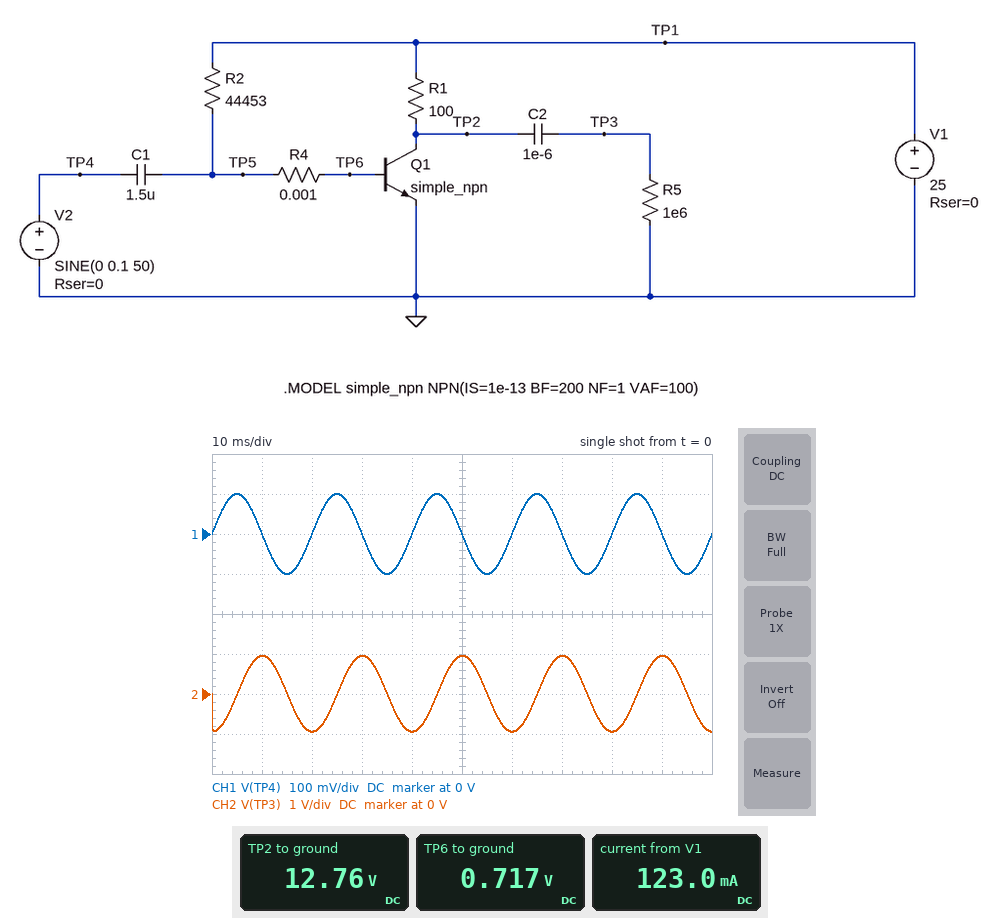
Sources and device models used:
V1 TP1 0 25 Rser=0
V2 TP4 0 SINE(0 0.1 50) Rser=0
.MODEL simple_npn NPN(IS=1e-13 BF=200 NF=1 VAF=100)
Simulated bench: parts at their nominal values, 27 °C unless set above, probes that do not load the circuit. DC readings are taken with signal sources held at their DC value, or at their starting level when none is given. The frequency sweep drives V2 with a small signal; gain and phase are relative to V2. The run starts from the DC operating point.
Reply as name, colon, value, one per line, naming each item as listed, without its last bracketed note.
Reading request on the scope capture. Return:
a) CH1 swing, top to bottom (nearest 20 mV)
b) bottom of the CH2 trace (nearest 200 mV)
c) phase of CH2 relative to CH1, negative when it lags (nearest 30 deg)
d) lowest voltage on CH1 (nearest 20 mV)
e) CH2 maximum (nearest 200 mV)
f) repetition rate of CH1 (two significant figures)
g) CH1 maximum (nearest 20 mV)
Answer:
CH1 swing, top to bottom: 200 mV
bottom of the CH2 trace: -1.0 V
phase of CH2 relative to CH1, negative when it lags: -90 deg
lowest voltage on CH1: -100 mV
CH2 maximum: 1.0 V
repetition rate of CH1: 50 Hz
CH1 maximum: 100 mV
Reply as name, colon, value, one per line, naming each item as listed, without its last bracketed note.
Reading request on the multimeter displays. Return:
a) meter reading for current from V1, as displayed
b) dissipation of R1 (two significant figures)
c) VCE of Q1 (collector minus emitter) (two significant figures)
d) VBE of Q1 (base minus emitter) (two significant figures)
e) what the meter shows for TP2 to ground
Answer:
meter reading for current from V1, as displayed: 123.0 mA
dissipation of R1: 1.5 W
VCE of Q1 (collector minus emitter): 13 V
VBE of Q1 (base minus emitter): 720 mV
what the meter shows for TP2 to ground: 12.76 V
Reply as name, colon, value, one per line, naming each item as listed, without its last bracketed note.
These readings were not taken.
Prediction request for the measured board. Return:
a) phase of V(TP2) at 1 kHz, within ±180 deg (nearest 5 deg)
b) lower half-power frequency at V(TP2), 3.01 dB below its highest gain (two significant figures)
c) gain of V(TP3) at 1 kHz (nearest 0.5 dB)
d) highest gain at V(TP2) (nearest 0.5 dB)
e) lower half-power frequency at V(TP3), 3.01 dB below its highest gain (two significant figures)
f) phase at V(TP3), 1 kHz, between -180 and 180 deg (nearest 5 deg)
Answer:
phase of V(TP2) at 1 kHz, within ±180 deg: -115 deg
lower half-power frequency at V(TP2), 3.01 dB below its highest gain: 2.2 kHz
gain of V(TP3) at 1 kHz: 45.0 dB
highest gain at V(TP2): 52.5 dB
lower half-power frequency at V(TP3), 3.01 dB below its highest gain: 2.2 kHz
phase at V(TP3), 1 kHz, between -180 and 180 deg: -115 deg
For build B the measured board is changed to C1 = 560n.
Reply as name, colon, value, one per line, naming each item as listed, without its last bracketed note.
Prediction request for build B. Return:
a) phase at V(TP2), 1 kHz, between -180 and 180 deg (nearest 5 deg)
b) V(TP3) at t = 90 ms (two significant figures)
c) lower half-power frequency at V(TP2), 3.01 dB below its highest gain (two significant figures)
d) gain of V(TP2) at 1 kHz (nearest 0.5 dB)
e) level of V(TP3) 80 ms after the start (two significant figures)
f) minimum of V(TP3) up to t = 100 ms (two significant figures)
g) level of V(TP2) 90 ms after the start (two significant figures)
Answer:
phase at V(TP2), 1 kHz, between -180 and 180 deg: -100 deg
V(TP3) at t = 90 ms: 360 mV
lower half-power frequency at V(TP2), 3.01 dB below its highest gain: 6.0 kHz
gain of V(TP2) at 1 kHz: 37.0 dB
level of V(TP3) 80 ms after the start: -350 mV
minimum of V(TP3) up to t = 100 ms: -360 mV
level of V(TP2) 90 ms after the start: 13 V
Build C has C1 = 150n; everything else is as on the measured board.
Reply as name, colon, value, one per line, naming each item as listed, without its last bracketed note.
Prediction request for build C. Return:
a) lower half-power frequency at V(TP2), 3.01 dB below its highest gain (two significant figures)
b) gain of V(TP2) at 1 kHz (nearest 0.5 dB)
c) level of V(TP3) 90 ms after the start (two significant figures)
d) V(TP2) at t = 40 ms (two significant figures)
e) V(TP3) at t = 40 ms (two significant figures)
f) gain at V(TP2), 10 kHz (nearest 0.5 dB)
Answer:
lower half-power frequency at V(TP2), 3.01 dB below its highest gain: 22 kHz
gain of V(TP2) at 1 kHz: 25.5 dB
level of V(TP3) 90 ms after the start: 95 mV
V(TP2) at t = 40 ms: 13 V
V(TP3) at t = 40 ms: -95 mV
gain at V(TP2), 10 kHz: 45.0 dB
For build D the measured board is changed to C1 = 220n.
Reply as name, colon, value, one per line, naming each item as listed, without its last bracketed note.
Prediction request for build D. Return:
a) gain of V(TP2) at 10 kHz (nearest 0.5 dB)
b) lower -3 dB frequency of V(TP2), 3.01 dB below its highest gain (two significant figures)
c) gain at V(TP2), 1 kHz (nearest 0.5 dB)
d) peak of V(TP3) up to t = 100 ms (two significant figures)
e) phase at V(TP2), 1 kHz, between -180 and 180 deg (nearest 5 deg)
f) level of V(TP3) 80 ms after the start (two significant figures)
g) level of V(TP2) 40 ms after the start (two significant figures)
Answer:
gain of V(TP2) at 10 kHz: 47.5 dB
lower -3 dB frequency of V(TP2), 3.01 dB below its highest gain: 15 kHz
gain at V(TP2), 1 kHz: 29.0 dB
peak of V(TP3) up to t = 100 ms: 140 mV
phase at V(TP2), 1 kHz, between -180 and 180 deg: -95 deg
level of V(TP3) 80 ms after the start: -140 mV
level of V(TP2) 40 ms after the start: 13 V
